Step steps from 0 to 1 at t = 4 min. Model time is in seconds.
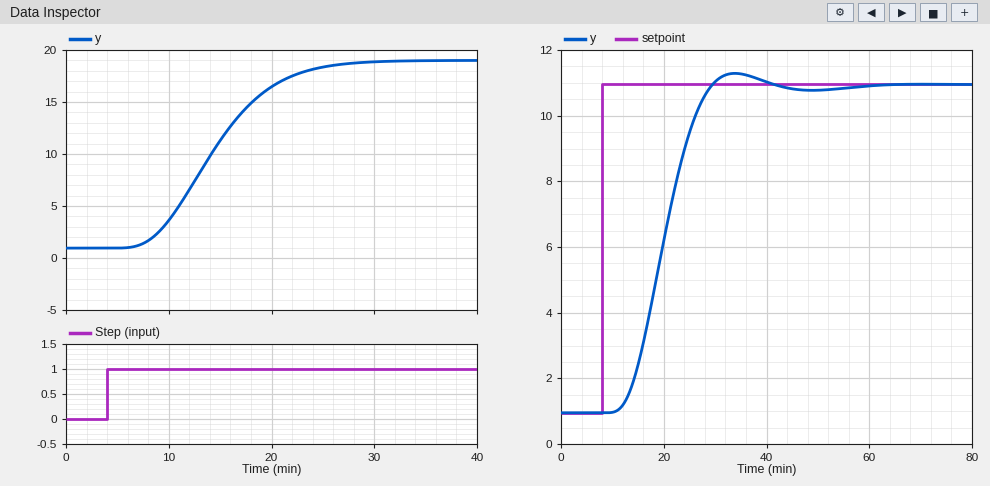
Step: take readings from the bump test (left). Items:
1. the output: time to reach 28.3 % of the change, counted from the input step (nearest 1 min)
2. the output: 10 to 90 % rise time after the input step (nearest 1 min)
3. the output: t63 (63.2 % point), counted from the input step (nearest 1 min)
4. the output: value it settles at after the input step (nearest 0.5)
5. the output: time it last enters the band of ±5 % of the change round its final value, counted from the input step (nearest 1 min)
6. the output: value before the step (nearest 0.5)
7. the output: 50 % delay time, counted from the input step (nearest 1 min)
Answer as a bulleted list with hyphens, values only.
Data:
- 8 min
- 12 min
- 12 min
- 19.0
- 20 min
- 1.0
- 10 min
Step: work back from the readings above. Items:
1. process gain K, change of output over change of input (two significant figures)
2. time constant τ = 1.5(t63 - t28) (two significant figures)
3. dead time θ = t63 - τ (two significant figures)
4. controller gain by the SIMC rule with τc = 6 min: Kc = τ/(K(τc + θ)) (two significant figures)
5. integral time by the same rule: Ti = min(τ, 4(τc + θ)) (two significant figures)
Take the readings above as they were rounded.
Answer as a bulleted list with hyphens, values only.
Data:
- 18
- 6.0 min
- 6.0 min
- 0.028
- 6.0 min
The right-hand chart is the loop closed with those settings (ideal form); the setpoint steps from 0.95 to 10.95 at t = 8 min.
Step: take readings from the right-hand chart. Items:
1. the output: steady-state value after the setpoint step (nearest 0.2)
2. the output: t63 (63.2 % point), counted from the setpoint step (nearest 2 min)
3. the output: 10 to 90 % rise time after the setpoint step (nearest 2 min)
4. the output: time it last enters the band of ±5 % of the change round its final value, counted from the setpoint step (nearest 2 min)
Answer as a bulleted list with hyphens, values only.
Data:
- 11.0
- 14 min
- 12 min
- 20 min
